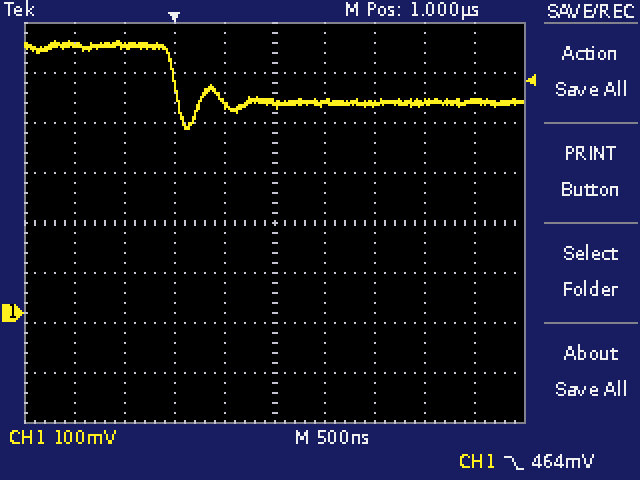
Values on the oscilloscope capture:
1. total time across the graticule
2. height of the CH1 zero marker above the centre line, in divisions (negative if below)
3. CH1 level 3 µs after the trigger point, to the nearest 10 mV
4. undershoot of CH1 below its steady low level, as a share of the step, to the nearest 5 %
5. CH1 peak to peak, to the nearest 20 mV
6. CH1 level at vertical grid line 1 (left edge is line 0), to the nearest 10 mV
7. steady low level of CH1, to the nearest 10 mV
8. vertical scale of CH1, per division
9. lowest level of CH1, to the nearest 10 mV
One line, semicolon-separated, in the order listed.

5 µs; -1.8 div; 420 mV; 45 %; 180 mV; 540 mV; 420 mV; 100 mV; 370 mV
